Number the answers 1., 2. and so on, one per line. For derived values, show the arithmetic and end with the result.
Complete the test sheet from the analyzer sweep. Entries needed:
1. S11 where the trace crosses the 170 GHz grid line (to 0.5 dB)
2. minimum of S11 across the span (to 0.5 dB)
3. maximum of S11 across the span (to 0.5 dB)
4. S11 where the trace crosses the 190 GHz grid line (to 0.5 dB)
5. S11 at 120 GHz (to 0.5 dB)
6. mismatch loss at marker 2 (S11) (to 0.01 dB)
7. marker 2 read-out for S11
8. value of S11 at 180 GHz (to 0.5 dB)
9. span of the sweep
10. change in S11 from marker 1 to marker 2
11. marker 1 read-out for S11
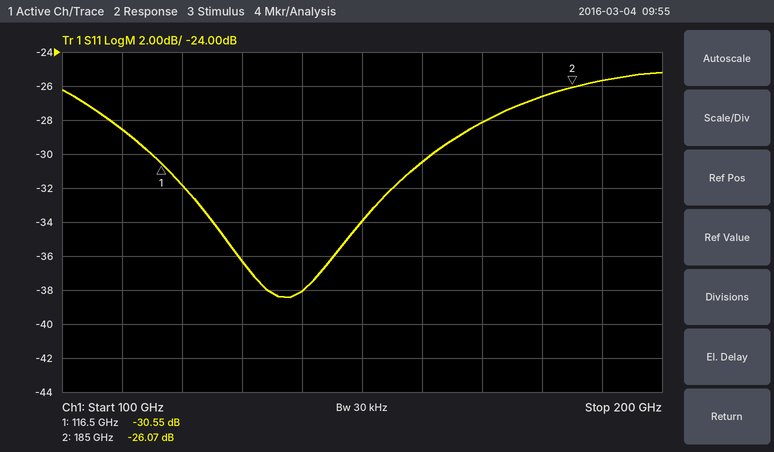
1. -28.0 dB
2. -38.5 dB
3. -25.0 dB
4. -25.5 dB
5. -32.0 dB
6. −10 log10(1 − 10^(-26.07/10)) ≈ 0.01 dB
7. -26.07 dB
8. -26.5 dB
9. 100 GHz
10. -26.07 − (-30.55) = 4.48 dB
11. -30.55 dB
